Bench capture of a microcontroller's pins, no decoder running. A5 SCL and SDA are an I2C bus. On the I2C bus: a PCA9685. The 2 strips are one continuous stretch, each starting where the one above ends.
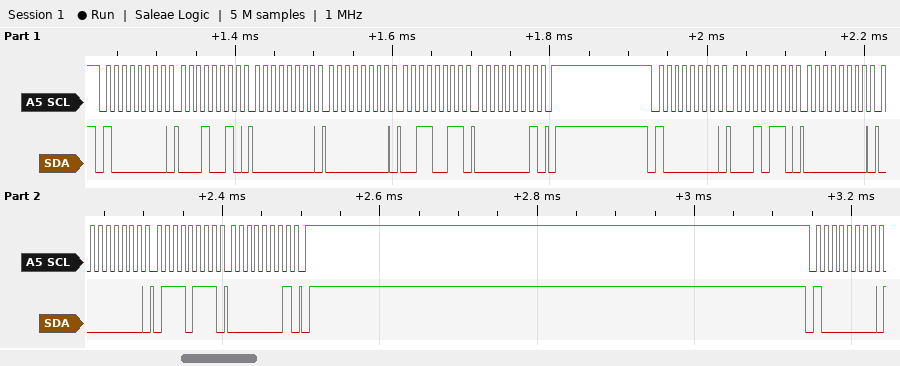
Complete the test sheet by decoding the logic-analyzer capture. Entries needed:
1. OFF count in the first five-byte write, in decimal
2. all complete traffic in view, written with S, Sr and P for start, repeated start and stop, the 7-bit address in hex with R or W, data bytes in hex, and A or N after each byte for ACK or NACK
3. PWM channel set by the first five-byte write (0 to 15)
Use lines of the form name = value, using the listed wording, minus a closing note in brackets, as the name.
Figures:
OFF count in the first five-byte write, in decimal = 307
all complete traffic in view, written with S, Sr and P for start, repeated start and stop, the 7-bit address in hex with R or W, data bytes in hex, and A or N after each byte for ACK or NACK = S 40W A 12 A 00 A 00 A 33 A 01 A P S 40W A 16 A 00 A 00 A 77 A 01 A P S 40W A
PWM channel set by the first five-byte write = 3
